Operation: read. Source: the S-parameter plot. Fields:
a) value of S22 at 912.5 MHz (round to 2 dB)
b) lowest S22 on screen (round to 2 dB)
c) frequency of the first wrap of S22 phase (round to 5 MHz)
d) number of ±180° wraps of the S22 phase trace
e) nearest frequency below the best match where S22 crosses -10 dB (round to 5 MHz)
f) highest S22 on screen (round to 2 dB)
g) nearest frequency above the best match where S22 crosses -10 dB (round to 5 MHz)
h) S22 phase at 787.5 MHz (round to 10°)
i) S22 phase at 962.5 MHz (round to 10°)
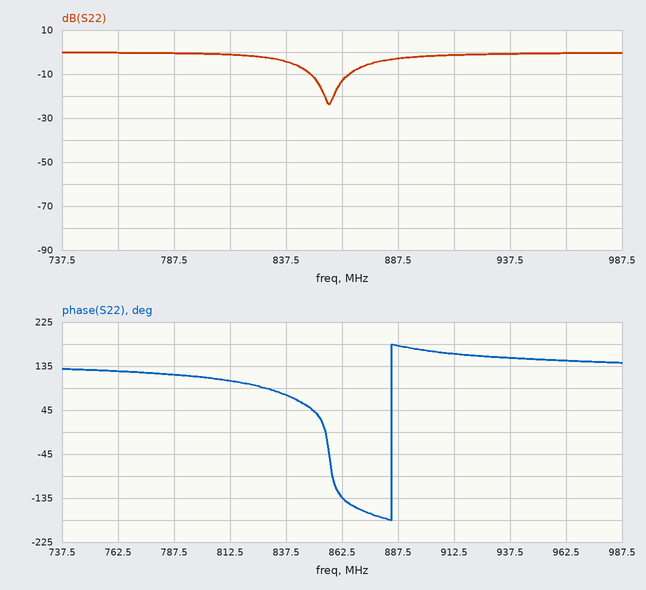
-2 dB
-24 dB
885 MHz
1
850 MHz
0 dB
865 MHz
120°
150°
